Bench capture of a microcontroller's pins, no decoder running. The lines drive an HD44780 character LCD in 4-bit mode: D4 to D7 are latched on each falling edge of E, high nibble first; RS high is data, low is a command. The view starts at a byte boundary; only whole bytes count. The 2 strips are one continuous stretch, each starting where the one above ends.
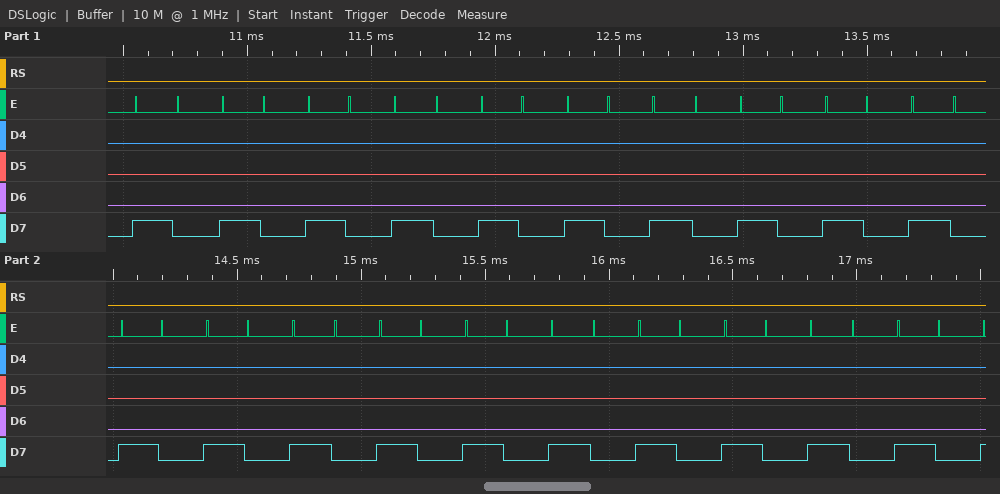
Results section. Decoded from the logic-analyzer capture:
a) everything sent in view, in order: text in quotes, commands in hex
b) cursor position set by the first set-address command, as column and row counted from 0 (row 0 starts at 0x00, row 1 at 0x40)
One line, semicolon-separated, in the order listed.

0x80 0x80 0x80 0x80 0x80 0x80 0x80 0x80 0x80 0x80 0x80 0x80 0x80 0x80 0x80 0x80 0x80 0x80 0x80 0x80; column 0, row 0
